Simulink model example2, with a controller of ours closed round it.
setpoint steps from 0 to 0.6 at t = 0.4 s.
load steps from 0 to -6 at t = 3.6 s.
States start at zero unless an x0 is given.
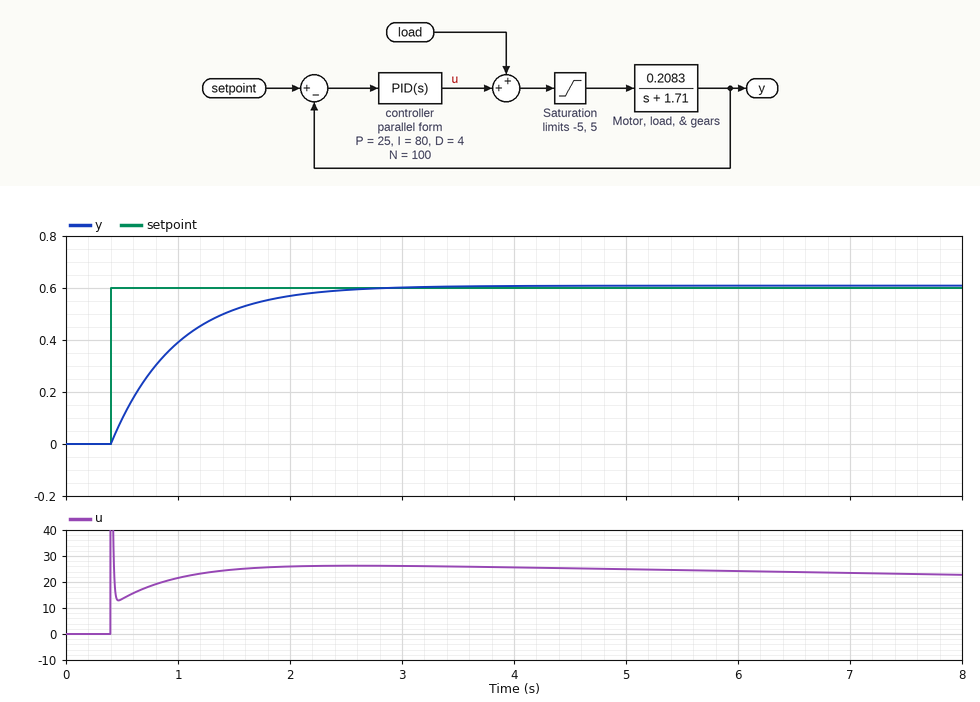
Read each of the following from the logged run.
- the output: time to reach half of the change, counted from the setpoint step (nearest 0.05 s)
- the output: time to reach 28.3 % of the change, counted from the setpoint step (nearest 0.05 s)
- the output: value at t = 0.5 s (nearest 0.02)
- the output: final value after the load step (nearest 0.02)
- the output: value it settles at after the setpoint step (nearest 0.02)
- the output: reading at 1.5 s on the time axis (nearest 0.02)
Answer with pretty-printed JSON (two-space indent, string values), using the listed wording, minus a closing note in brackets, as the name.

{
  "the output: time to reach half of the change, counted from the setpoint step": "0.40 s",
  "the output: time to reach 28.3 % of the change, counted from the setpoint step": "0.20 s",
  "the output: value at t = 0.5 s": "0.10",
  "the output: final value after the load step": "0.60",
  "the output: value it settles at after the setpoint step": "0.60",
  "the output: reading at 1.5 s on the time axis": "0.52"
}
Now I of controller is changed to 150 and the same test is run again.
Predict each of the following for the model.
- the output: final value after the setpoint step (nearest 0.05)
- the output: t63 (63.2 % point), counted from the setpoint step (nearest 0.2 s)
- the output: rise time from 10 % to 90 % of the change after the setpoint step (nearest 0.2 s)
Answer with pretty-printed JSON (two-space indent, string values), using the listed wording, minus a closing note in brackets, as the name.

{
  "the output: final value after the setpoint step": "0.60",
  "the output: t63 (63.2 % point), counted from the setpoint step": "0.6 s",
  "the output: rise time from 10 % to 90 % of the change after the setpoint step": "1.2 s"
}
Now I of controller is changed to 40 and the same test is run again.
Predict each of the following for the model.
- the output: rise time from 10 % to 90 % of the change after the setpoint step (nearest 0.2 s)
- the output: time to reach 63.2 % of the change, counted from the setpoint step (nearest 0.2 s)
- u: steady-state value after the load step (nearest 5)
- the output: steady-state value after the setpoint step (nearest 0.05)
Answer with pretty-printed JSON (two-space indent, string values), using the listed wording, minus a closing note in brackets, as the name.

{
  "the output: rise time from 10 % to 90 % of the change after the setpoint step": "1.2 s",
  "the output: time to reach 63.2 % of the change, counted from the setpoint step": "0.6 s",
  "u: steady-state value after the load step": "10",
  "the output: steady-state value after the setpoint step": "0.60"
}
